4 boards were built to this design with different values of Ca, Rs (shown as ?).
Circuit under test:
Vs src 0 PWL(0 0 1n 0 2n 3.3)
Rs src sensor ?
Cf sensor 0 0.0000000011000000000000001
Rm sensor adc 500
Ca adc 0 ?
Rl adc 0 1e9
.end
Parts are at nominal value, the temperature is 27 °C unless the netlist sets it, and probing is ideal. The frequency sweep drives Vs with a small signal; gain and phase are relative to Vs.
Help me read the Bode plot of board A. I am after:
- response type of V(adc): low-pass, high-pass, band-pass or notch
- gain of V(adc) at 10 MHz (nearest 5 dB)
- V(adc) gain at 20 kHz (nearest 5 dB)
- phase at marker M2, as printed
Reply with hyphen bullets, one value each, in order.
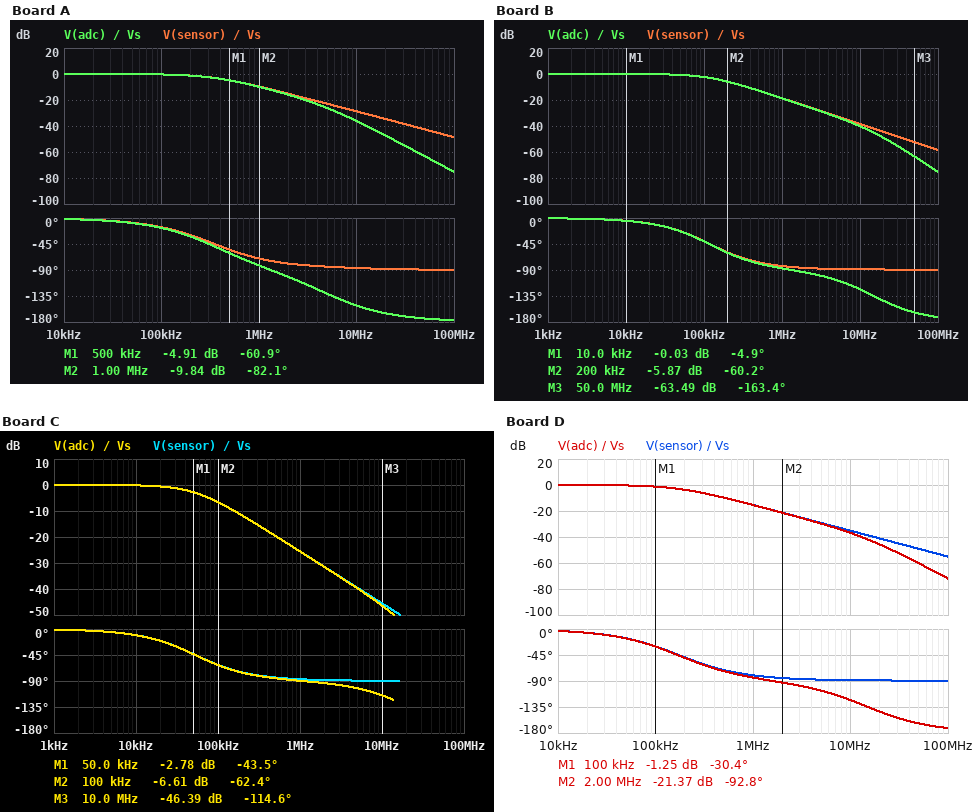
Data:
- low-pass
- -35 dB
- 0 dB
- -82.1 deg
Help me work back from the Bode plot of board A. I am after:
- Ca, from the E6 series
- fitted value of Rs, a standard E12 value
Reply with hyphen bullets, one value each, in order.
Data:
- 68 pF
- 390 Ω
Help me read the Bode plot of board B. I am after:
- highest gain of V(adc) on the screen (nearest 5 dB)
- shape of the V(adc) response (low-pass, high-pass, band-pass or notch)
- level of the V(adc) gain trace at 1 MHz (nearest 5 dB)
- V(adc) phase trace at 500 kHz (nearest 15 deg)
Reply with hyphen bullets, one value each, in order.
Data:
- 0 dB
- low-pass
- -20 dB
- -75 deg
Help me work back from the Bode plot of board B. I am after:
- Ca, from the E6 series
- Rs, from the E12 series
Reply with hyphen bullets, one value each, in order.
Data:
- 22 pF
- 1.2 kΩ
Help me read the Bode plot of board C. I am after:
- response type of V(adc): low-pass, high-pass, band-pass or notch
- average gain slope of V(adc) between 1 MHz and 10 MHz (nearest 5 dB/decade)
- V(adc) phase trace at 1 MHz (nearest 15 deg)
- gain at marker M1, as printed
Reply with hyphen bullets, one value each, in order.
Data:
- low-pass
- -20 dB/decade
- -90 deg
- -2.78 dB
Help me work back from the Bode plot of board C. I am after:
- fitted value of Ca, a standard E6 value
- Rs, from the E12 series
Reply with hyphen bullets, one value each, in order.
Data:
- 15 pF
- 2.7 kΩ
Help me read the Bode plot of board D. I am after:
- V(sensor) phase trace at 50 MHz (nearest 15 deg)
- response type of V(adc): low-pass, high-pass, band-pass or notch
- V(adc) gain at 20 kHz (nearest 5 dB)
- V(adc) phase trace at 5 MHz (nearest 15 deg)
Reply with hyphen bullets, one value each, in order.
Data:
- -90 deg
- low-pass
- 0 dB
- -105 deg
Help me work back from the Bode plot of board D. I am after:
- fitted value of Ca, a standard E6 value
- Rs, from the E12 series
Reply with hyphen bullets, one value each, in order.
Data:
- 22 pF
- 820 Ω
